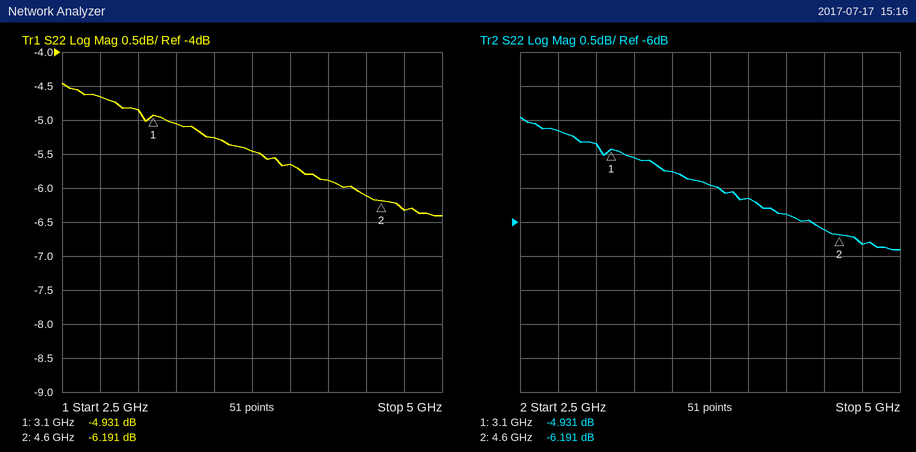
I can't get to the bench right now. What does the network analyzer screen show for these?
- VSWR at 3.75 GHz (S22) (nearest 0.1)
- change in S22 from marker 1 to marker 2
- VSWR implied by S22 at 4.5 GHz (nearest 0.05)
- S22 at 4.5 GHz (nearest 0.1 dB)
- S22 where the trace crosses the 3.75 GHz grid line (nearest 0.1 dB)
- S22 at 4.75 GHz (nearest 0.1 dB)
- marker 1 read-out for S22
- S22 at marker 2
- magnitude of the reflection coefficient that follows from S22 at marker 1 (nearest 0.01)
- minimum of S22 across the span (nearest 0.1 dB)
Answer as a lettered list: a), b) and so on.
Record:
a) 3.3
b) -1.260 dB
c) 2.95
d) -6.1 dB
e) -5.5 dB
f) -6.3 dB
g) -4.931 dB
h) -6.191 dB
i) 0.57
j) -6.4 dB
